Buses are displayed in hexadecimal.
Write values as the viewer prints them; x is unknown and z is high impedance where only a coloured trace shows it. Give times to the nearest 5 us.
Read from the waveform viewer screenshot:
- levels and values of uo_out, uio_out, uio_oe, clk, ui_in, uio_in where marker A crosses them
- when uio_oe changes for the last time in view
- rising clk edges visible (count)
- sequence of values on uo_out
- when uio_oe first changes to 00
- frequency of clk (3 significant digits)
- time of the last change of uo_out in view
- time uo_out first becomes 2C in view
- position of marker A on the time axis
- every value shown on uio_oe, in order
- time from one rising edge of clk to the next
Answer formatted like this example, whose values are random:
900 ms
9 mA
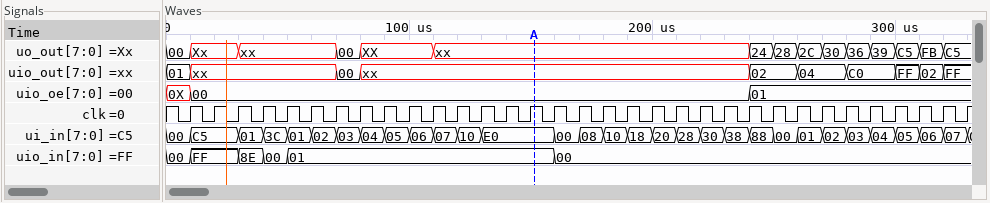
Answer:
uo_out=xx, uio_out=xx, uio_oe=00, clk=1, ui_in=E0, uio_in=01
240 us
33
00, Xx, xx, 00, XX, xx, 24, 28, 2C, 30, 36, 39, C5, FB, C5
10 us
100 kHz
320 us
260 us
150 us
0X, 00, 01
10 us
